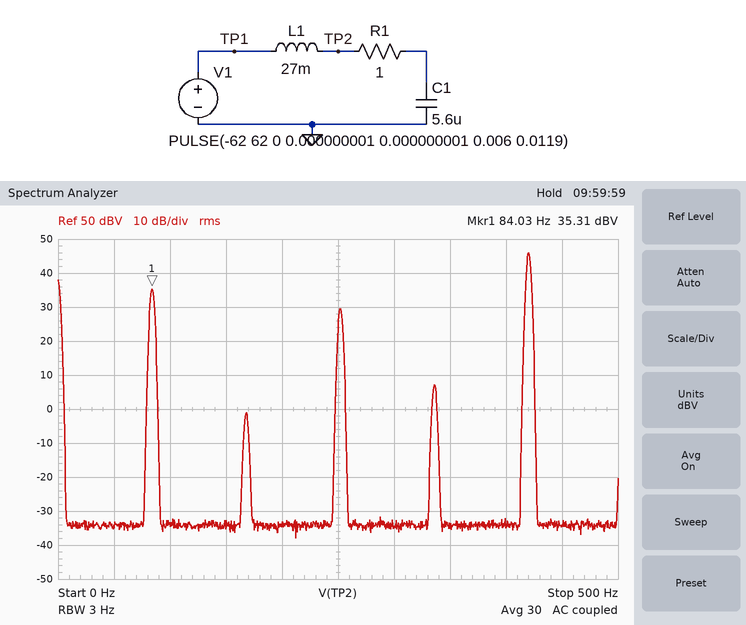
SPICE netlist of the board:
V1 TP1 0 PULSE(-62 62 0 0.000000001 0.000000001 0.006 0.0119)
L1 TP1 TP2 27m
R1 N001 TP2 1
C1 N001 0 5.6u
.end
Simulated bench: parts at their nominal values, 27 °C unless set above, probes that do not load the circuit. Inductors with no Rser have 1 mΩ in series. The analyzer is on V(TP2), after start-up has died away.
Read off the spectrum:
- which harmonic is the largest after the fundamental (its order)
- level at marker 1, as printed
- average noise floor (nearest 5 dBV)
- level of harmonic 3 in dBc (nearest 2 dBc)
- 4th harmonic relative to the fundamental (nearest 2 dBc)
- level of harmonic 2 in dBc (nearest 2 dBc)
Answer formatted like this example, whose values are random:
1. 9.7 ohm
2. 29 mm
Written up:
1. 5
2. 35.31 dBV
3. -35 dBV
4. -6 dBc
5. -28 dBc
6. -36 dBc
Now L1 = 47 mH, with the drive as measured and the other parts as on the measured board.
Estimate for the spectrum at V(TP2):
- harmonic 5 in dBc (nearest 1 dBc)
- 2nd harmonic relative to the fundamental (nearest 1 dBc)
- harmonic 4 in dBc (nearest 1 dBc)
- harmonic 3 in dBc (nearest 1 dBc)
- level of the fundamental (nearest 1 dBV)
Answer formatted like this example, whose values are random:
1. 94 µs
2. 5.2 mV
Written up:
1. -13 dBc
2. -35 dBc
3. -23 dBc
4. -1 dBc
5. 36 dBV
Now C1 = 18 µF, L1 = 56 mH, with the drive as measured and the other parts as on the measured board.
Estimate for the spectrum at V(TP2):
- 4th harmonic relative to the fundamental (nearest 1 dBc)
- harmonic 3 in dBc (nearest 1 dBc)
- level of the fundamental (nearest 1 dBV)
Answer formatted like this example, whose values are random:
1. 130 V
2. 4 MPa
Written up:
1. -51 dBc
2. -16 dBc
3. 38 dBV
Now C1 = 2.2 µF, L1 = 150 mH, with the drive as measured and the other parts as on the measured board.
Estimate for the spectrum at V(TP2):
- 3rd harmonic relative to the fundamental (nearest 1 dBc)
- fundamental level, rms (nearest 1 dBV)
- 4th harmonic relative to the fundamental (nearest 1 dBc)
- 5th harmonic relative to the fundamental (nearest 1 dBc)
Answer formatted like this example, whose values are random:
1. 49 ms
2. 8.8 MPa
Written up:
1. 5 dBc
2. 36 dBV
3. -32 dBc
4. -17 dBc
